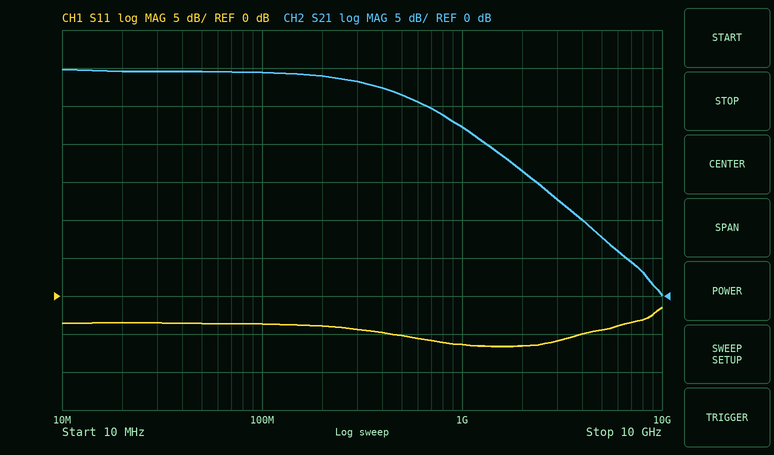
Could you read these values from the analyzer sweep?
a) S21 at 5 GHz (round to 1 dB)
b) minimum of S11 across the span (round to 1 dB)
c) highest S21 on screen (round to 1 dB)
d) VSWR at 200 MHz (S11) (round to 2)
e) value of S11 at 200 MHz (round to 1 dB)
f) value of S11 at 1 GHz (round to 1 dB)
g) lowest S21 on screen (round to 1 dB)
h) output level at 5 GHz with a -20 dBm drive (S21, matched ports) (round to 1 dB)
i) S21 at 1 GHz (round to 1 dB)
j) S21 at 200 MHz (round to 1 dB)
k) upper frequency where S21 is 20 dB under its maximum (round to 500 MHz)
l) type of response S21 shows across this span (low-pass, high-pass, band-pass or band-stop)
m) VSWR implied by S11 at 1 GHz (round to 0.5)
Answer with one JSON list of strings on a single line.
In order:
["8 dB", "-7 dB", "30 dB", "4", "-4 dB", "-6 dB", "0 dB", "-12 dBm", "22 dB", "29 dB", "4.0 GHz", "low-pass", "3.0"]
